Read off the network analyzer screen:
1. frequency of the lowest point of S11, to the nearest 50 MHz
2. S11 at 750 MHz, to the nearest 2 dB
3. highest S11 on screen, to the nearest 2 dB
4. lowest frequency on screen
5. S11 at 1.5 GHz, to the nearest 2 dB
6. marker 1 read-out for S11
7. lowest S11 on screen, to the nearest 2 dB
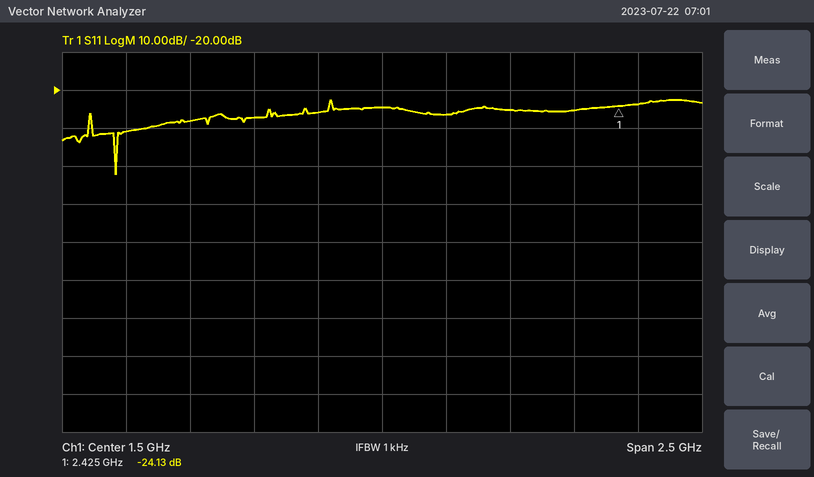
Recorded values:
450 MHz
-28 dB
-22 dB
250 MHz
-24 dB
-24.13 dB
-42 dB
